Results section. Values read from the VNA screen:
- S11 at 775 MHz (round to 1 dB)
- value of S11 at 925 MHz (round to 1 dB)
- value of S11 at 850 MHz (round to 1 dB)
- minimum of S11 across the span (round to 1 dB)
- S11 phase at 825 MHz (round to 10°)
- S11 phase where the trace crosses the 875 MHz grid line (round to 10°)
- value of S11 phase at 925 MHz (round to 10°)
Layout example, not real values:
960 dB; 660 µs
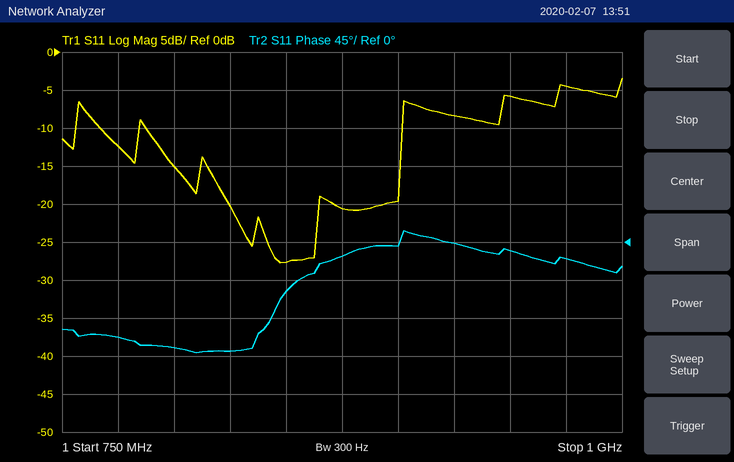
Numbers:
-12 dB; -8 dB; -28 dB; -28 dB; -130°; -20°; 0°
